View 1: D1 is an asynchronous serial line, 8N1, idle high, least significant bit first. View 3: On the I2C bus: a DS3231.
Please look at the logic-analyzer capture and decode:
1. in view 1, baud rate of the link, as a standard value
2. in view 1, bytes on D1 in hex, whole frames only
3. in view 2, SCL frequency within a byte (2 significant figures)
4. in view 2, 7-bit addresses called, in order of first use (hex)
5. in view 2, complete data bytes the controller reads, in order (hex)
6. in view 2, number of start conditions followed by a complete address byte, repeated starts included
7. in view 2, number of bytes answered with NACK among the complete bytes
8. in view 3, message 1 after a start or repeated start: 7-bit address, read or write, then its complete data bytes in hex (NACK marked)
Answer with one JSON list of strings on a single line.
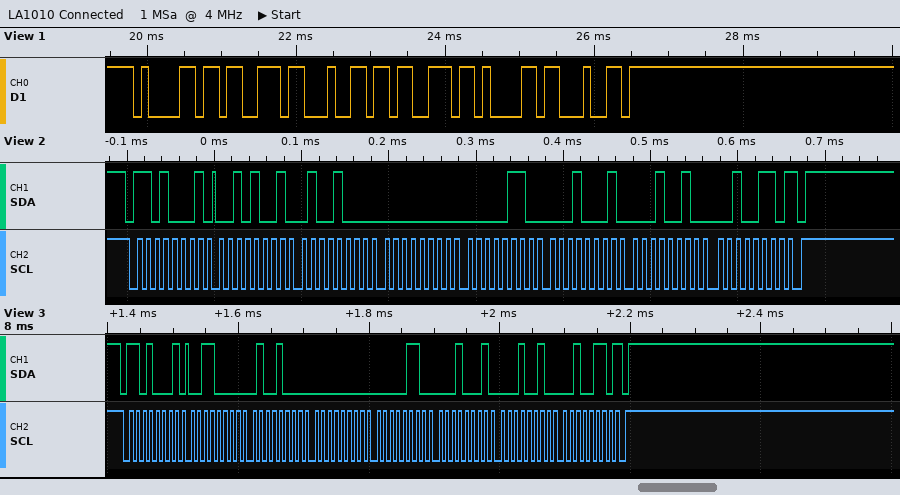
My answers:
["9600 baud", "61 73 64 73 61 64", "100 kHz", "0x68", "29 48 00 06 11 12 26", "1", "1", "0x68 read: 30 48 00 06 11 12 26 NACK"]
